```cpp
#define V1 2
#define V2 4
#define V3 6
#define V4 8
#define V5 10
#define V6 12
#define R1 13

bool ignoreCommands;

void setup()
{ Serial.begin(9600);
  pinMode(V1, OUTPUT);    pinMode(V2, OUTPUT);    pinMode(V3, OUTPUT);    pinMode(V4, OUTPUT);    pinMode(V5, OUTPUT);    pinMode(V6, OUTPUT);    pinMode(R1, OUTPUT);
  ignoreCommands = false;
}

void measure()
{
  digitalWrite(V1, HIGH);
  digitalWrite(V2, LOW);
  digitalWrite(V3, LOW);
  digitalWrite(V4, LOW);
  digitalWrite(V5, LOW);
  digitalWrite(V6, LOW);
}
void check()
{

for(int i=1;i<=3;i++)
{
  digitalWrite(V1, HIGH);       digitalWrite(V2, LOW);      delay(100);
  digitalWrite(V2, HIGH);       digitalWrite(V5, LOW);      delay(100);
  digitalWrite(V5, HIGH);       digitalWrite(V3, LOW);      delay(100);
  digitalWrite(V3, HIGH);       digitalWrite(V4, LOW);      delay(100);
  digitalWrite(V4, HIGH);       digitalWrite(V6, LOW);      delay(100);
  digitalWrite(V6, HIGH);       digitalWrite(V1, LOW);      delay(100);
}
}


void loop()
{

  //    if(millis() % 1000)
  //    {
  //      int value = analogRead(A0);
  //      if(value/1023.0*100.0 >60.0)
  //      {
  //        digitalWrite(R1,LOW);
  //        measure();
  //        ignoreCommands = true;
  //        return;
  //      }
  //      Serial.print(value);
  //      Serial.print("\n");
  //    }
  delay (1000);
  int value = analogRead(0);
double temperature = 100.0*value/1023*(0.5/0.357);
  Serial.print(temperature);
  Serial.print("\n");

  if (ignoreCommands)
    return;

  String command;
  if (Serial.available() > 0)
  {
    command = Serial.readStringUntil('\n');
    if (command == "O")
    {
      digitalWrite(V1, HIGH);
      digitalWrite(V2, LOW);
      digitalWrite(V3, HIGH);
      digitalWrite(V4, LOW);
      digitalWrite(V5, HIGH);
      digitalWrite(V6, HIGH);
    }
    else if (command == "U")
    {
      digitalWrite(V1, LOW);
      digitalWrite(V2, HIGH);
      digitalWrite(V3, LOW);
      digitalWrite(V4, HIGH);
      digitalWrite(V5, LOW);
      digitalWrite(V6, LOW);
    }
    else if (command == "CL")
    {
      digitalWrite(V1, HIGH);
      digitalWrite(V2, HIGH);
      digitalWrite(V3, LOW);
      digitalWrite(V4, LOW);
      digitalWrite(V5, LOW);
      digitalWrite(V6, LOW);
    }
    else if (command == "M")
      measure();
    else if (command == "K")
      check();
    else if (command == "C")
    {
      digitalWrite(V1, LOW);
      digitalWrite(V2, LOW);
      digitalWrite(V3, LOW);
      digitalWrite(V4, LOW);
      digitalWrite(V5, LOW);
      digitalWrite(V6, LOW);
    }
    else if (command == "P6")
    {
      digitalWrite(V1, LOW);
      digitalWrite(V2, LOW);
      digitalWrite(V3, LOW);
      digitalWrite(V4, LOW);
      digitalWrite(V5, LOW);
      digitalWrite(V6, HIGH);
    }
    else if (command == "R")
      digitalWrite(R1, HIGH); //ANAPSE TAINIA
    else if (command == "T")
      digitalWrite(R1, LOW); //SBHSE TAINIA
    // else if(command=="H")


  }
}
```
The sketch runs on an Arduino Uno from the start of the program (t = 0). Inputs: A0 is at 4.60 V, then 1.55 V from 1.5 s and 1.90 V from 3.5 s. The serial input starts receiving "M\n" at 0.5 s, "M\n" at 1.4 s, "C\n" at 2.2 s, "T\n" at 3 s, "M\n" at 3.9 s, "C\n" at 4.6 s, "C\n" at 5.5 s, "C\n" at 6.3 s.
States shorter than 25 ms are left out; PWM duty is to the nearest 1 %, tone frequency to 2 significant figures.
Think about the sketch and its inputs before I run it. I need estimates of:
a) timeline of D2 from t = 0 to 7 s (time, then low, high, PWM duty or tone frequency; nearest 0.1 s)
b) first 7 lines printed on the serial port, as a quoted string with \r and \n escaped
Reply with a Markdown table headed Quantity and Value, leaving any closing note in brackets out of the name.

| Quantity | Value |
|---|---|
| timeline of D2 from t = 0 to 7 s | 0 s low; 1 s high; 3 s low; 5 s high; 6 s low |
| first 7 lines printed on the serial port, as a quoted string with \r and \n escaped | "128.97\n43.40\n43.40\n53.26\n53.26\n53.26\n53.26\n" |
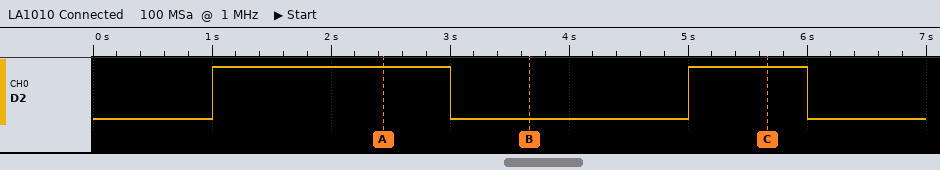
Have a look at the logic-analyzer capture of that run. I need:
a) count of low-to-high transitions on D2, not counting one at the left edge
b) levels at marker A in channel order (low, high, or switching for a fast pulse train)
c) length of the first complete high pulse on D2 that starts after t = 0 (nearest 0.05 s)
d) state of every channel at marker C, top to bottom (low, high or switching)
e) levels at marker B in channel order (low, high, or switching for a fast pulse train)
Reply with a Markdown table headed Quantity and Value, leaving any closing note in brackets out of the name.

| Quantity | Value |
|---|---|
| count of low-to-high transitions on D2, not counting one at the left edge | 2 |
| levels at marker A in channel order | D2 high |
| length of the first complete high pulse on D2 that starts after t = 0 | 2.00 s |
| state of every channel at marker C, top to bottom | D2 high |
| levels at marker B in channel order | D2 low |
